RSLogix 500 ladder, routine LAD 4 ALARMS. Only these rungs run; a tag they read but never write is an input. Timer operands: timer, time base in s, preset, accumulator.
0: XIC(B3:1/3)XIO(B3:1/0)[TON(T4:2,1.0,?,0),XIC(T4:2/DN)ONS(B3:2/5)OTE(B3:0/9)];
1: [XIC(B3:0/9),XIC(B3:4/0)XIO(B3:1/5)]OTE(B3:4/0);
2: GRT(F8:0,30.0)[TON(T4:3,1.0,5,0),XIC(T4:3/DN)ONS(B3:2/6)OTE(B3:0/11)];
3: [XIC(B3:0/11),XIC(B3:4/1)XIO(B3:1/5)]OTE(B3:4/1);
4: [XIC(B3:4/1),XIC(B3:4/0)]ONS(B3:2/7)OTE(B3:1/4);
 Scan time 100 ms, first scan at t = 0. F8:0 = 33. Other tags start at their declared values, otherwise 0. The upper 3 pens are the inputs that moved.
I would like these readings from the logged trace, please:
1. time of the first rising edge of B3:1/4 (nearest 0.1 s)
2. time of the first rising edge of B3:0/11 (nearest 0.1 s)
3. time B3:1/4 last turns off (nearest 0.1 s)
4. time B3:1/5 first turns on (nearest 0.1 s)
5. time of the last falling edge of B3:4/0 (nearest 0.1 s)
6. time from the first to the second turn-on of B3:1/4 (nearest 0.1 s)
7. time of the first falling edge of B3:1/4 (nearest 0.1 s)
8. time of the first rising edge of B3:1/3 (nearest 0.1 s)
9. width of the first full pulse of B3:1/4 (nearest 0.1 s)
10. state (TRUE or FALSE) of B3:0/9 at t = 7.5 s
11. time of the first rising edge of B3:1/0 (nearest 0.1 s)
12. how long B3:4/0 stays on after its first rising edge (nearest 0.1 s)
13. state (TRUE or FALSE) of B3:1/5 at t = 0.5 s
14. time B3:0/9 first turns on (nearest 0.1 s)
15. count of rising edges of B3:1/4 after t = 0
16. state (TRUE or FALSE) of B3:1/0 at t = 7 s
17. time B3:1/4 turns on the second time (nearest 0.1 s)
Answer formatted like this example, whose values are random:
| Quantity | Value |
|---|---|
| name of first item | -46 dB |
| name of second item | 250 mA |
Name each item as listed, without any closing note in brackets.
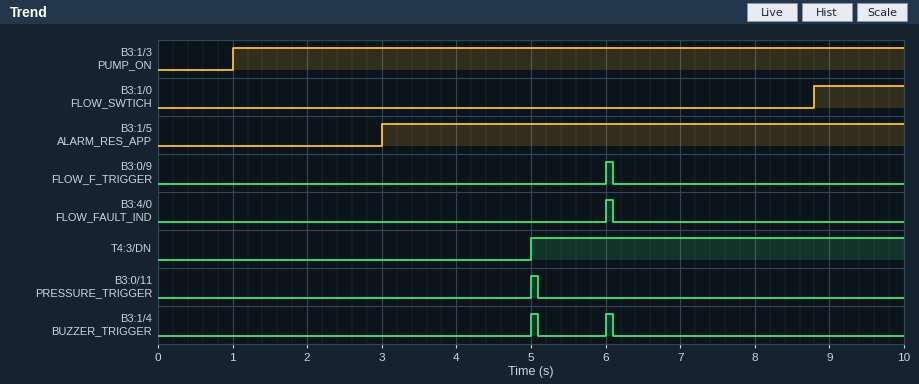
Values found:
| Quantity | Value |
|---|---|
| time of the first rising edge of B3:1/4 | 5.0 s |
| time of the first rising edge of B3:0/11 | 5.0 s |
| time B3:1/4 last turns off | 6.1 s |
| time B3:1/5 first turns on | 3.0 s |
| time of the last falling edge of B3:4/0 | 6.1 s |
| time from the first to the second turn-on of B3:1/4 | 1.0 s |
| time of the first falling edge of B3:1/4 | 5.1 s |
| time of the first rising edge of B3:1/3 | 1.0 s |
| width of the first full pulse of B3:1/4 | 0.1 s |
| state (TRUE or FALSE) of B3:0/9 at t = 7.5 s | FALSE |
| time of the first rising edge of B3:1/0 | 8.8 s |
| how long B3:4/0 stays on after its first rising edge | 0.1 s |
| state (TRUE or FALSE) of B3:1/5 at t = 0.5 s | FALSE |
| time B3:0/9 first turns on | 6.0 s |
| count of rising edges of B3:1/4 after t = 0 | 2 |
| state (TRUE or FALSE) of B3:1/0 at t = 7 s | FALSE |
| time B3:1/4 turns on the second time | 6.0 s |
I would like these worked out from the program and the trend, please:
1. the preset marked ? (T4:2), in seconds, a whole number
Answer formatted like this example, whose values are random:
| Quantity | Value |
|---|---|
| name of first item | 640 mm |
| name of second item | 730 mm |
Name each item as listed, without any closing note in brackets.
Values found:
| Quantity | Value |
|---|---|
| the preset marked ? (T4:2), in seconds, a whole number | 5 s |
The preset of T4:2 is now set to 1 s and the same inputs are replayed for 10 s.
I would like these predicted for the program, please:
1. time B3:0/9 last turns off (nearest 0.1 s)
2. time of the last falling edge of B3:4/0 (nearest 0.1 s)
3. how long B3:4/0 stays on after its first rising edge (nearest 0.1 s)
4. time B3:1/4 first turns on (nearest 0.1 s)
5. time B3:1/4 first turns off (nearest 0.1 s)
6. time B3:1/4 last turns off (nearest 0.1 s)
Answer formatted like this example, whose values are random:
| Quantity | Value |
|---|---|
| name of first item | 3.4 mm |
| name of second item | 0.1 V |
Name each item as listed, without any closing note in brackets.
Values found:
| Quantity | Value |
|---|---|
| time B3:0/9 last turns off | 2.1 s |
| time of the last falling edge of B3:4/0 | 3.0 s |
| how long B3:4/0 stays on after its first rising edge | 1.0 s |
| time B3:1/4 first turns on | 2.0 s |
| time B3:1/4 first turns off | 2.1 s |
| time B3:1/4 last turns off | 5.1 s |
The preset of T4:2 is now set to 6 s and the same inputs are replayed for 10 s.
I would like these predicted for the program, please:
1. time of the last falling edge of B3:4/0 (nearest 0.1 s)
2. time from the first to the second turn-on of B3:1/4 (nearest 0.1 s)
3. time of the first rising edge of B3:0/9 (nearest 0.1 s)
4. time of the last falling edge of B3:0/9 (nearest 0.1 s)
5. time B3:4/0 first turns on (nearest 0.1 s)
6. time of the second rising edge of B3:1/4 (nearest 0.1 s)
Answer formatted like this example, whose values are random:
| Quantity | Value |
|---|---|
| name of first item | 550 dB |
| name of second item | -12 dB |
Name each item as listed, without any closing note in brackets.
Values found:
| Quantity | Value |
|---|---|
| time of the last falling edge of B3:4/0 | 7.1 s |
| time from the first to the second turn-on of B3:1/4 | 2.0 s |
| time of the first rising edge of B3:0/9 | 7.0 s |
| time of the last falling edge of B3:0/9 | 7.1 s |
| time B3:4/0 first turns on | 7.0 s |
| time of the second rising edge of B3:1/4 | 7.0 s |
